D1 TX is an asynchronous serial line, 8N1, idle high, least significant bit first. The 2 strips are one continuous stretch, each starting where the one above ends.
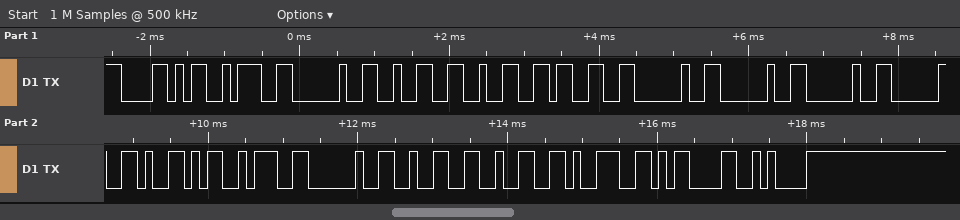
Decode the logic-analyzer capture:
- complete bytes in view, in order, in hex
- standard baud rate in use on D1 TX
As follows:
58 3A 20 32 32 33 20 20 20 20 59 3A 20 32 32 39 0D 0A
9600 baud
